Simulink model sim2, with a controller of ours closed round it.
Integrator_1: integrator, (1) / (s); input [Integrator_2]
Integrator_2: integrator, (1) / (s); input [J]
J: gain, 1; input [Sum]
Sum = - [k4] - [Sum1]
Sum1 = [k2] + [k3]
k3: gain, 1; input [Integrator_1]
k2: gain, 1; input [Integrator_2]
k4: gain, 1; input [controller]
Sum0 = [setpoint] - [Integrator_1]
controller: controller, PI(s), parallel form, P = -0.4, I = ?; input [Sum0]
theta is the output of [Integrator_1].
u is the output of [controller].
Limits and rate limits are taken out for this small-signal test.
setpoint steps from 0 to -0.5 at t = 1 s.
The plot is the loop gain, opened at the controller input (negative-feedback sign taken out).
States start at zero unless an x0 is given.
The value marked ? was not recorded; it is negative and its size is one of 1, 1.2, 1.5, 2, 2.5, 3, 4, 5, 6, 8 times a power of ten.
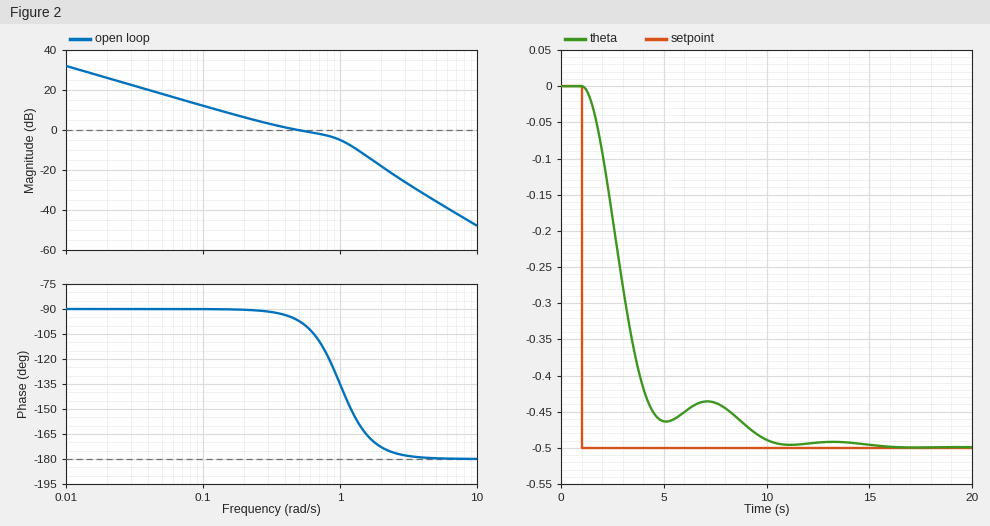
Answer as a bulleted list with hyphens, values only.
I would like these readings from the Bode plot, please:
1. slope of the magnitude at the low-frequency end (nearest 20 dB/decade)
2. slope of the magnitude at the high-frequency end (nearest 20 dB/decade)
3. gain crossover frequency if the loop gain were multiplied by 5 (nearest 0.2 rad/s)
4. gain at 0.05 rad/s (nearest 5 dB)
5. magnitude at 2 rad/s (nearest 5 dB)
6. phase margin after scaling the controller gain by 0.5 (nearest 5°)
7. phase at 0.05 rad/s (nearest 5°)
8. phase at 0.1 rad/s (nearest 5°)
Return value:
- -20 dB/decade
- -40 dB/decade
- 1.6 rad/s
- 20 dB
- -20 dB
- 90°
- -90°
- -90°
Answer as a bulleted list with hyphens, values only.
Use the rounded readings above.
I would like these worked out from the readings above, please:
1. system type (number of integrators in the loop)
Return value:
- 1
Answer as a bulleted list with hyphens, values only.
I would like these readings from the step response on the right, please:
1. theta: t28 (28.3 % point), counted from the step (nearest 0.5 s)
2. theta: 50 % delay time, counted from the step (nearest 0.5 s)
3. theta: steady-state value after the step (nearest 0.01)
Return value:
- 1.5 s
- 2.0 s
- -0.50
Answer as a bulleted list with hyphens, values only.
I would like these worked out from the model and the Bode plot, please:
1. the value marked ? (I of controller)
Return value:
- -0.4
